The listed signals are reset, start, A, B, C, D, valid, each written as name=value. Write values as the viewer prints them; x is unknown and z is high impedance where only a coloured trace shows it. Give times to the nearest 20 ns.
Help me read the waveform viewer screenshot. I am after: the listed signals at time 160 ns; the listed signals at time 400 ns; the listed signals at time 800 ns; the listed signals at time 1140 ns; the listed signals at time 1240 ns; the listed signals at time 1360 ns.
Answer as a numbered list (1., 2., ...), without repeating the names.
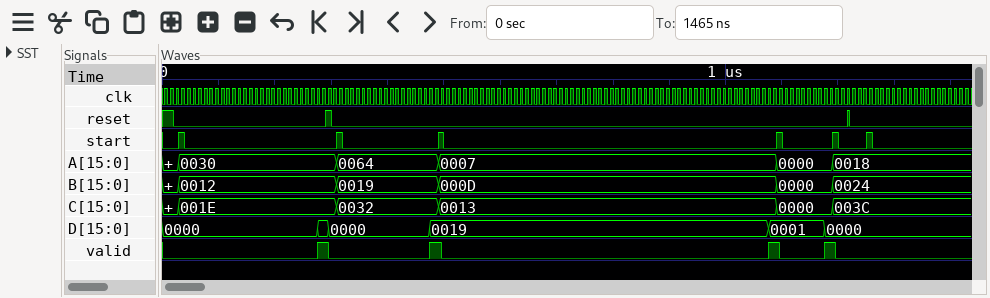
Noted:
1. reset=0, start=0, A=0030, B=0012, C=001E, D=0000, valid=0
2. reset=0, start=0, A=0064, B=0019, C=0032, D=0000, valid=0
3. reset=0, start=0, A=0007, B=000D, C=0013, D=0019, valid=0
4. reset=0, start=0, A=0000, B=0000, C=0000, D=0001, valid=0
5. reset=0, start=0, A=0018, B=0024, C=003C, D=0000, valid=0
6. reset=0, start=0, A=0018, B=0024, C=003C, D=0000, valid=0
